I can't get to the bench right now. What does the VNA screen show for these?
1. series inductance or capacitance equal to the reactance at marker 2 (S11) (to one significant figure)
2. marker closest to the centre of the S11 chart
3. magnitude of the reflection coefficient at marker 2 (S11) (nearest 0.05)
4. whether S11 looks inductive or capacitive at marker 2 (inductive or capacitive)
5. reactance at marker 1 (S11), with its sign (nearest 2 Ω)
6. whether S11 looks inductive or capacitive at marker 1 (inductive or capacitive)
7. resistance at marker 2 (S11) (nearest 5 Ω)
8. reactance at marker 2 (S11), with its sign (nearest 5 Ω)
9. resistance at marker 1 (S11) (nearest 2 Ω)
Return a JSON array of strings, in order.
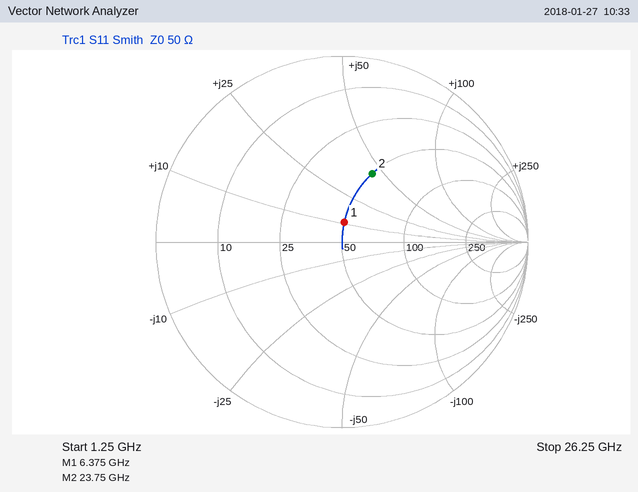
["300 pH", "marker 1", "0.40", "inductive", "+10 Ω", "inductive", "50 Ω", "+45 Ω", "50 Ω"]
